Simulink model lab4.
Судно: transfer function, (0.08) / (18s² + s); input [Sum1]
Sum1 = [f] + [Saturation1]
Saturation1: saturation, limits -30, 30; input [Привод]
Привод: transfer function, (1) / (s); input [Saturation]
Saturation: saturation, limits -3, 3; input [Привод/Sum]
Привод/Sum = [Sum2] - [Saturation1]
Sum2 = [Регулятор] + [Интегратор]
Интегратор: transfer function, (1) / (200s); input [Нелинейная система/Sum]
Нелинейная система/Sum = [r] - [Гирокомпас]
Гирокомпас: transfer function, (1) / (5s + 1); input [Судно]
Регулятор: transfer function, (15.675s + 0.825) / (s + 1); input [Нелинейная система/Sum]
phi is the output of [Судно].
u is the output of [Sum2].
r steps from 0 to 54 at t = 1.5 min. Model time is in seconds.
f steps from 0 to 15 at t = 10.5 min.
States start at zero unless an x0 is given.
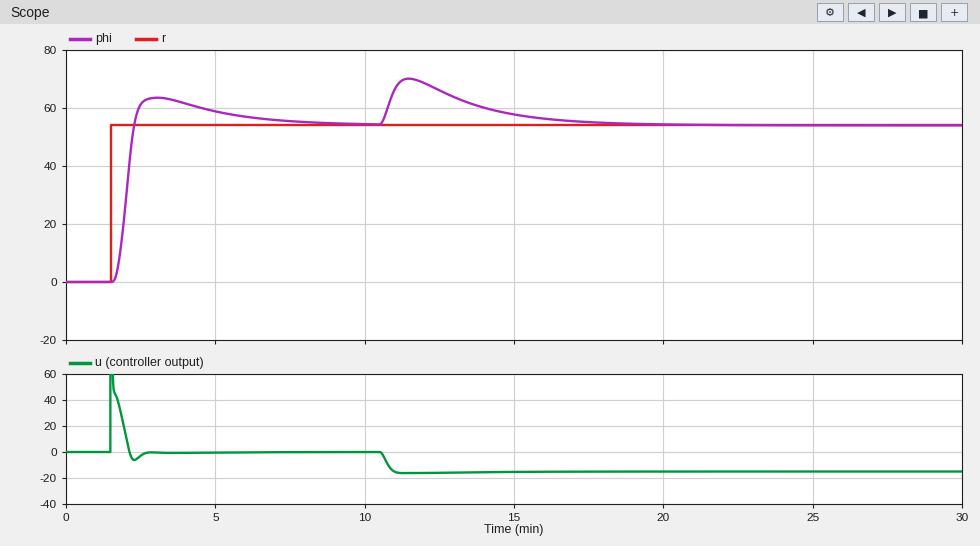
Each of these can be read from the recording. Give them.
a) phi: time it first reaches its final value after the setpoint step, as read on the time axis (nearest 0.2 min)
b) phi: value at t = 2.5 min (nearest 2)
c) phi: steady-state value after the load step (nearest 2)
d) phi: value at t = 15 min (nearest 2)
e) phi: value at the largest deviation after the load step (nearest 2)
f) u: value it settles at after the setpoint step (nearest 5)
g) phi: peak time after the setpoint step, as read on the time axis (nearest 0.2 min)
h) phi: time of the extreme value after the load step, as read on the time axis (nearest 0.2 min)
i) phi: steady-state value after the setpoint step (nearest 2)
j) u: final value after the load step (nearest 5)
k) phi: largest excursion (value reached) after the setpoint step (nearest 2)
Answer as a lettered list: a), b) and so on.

a) 2.2 min
b) 62
c) 54
d) 58
e) 70
f) 0
g) 3.0 min
h) 11.4 min
i) 54
j) -15
k) 64
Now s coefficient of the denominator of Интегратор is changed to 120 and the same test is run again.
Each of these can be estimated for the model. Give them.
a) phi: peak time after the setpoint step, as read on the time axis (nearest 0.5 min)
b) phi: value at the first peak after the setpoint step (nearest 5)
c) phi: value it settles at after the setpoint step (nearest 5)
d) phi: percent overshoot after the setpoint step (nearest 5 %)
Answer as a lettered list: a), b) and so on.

a) 2.5 min
b) 70
c) 55
d) 30 %
